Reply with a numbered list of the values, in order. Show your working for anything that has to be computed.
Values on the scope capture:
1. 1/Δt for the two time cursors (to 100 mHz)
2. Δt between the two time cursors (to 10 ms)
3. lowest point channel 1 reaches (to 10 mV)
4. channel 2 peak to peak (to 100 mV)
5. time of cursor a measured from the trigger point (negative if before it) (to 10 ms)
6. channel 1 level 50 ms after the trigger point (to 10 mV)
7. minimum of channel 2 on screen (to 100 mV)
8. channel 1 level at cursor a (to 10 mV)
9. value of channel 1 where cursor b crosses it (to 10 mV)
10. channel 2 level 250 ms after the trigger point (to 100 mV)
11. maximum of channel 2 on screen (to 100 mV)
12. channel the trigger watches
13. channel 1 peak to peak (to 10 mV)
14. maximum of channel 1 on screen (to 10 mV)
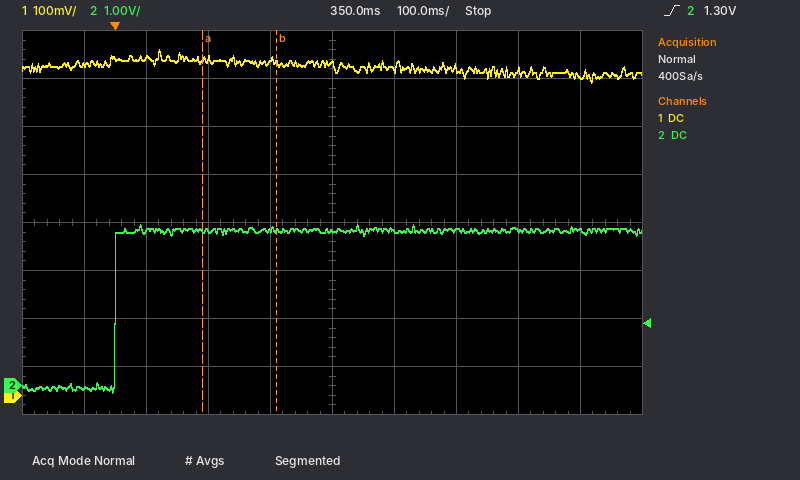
1. 1 / 120 ms ≈ 8.3 Hz
2. 120 ms
3. 650 mV
4. 3.4 V − (-100 mV) = 3.5 V
5. +140 ms
6. 700 mV
7. -100 mV
8. 700 mV
9. 690 mV
10. 3.3 V
11. 3.4 V
12. channel 2
13. 720 mV − (650 mV) = 70 mV
14. 720 mV
